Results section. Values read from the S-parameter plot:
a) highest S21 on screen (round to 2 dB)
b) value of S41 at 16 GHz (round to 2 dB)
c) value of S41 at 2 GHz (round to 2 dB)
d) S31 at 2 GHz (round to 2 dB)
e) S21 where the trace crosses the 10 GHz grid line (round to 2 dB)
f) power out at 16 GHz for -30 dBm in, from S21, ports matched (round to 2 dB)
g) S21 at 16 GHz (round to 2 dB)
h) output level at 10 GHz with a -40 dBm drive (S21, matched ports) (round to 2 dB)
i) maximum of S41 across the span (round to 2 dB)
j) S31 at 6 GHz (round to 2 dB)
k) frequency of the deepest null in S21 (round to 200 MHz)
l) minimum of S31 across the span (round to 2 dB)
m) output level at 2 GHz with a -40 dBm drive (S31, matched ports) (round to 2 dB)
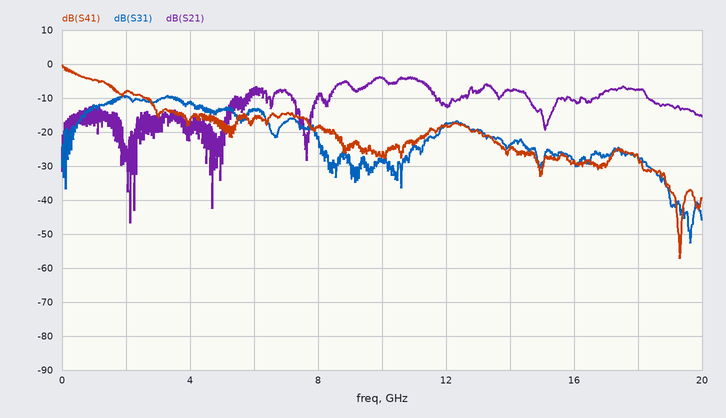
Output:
-4 dB
-28 dB
-8 dB
-10 dB
-4 dB
-40 dBm
-10 dB
-44 dBm
0 dB
-14 dB
2.2 GHz
-52 dB
-50 dBm
